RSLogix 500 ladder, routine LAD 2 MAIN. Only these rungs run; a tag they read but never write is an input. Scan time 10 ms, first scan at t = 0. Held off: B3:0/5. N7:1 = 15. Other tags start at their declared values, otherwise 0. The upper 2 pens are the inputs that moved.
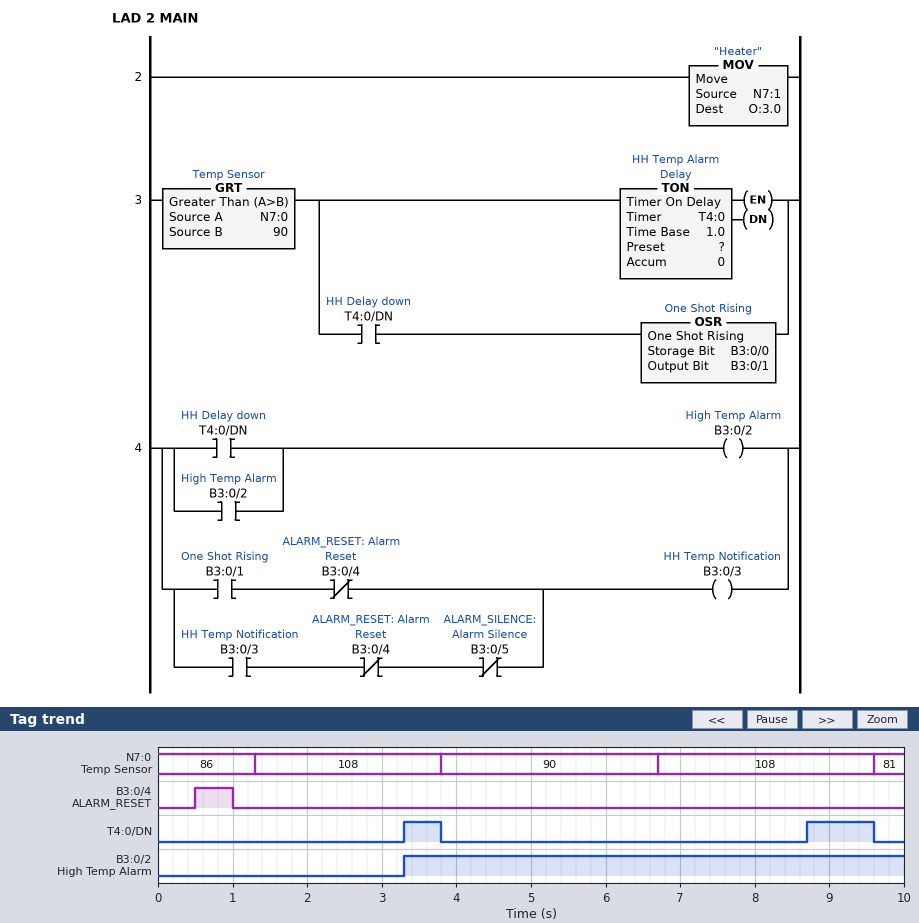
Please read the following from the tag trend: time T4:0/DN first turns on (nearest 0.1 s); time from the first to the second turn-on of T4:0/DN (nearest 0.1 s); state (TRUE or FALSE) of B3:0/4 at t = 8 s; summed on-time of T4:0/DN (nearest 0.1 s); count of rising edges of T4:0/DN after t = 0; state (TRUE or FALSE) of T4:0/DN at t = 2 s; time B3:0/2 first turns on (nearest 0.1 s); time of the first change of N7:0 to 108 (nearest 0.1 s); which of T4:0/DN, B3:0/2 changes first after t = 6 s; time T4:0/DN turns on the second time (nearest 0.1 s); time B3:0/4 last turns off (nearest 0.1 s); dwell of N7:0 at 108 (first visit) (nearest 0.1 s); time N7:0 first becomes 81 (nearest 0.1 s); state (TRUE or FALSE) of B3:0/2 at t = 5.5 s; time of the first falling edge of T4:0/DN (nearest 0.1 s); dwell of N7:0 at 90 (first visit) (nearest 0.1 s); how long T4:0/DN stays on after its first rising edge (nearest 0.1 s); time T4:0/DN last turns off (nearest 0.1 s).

3.3 s
5.4 s
FALSE
1.4 s
2
FALSE
3.3 s
1.3 s
T4:0/DN
8.7 s
1.0 s
2.5 s
9.6 s
TRUE
3.8 s
2.9 s
0.5 s
9.6 s
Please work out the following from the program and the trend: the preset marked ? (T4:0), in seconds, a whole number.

2 s
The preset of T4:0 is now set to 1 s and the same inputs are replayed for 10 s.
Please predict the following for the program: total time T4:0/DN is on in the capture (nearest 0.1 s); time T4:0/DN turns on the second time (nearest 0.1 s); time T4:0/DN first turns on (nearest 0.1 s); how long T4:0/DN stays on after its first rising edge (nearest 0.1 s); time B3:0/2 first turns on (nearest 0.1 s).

3.4 s
7.7 s
2.3 s
1.5 s
2.3 s
